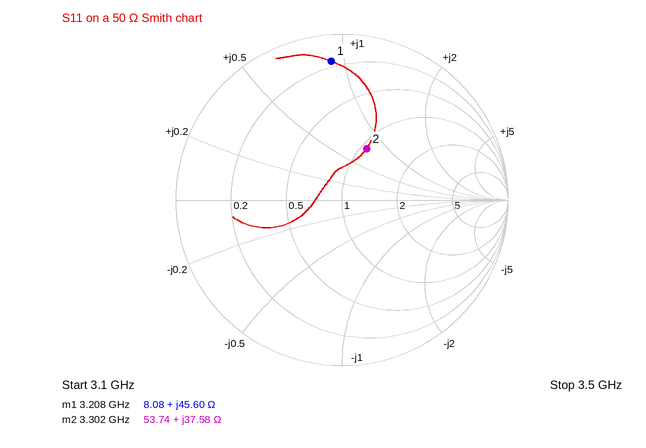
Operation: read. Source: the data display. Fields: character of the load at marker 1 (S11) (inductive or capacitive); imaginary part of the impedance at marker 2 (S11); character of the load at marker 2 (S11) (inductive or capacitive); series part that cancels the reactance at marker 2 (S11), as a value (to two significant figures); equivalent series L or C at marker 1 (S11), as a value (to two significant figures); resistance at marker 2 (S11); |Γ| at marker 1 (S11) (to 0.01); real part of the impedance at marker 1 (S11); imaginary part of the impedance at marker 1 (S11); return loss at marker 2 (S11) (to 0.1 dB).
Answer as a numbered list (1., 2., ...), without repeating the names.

1. inductive
2. +37.58 Ω
3. inductive
4. 1.3 pF
5. 2.3 nH
6. 53.74 Ω
7. 0.84
8. 8.08 Ω
9. +45.60 Ω
10. 9.3 dB
